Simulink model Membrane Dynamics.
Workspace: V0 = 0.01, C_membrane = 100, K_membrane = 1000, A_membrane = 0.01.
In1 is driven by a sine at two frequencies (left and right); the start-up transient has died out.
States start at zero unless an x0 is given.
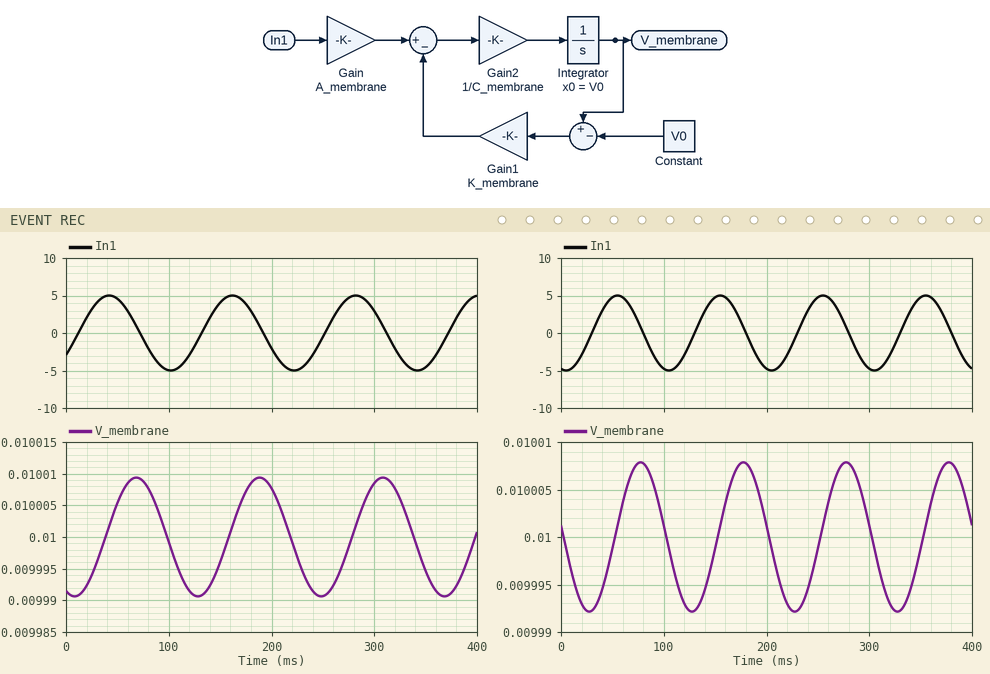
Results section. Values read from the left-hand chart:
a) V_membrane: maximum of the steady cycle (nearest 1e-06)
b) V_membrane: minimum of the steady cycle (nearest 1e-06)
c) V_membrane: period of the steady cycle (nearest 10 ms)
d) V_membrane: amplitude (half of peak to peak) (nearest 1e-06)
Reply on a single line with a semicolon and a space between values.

0.010009; 0.009991; 120 ms; 0.000009
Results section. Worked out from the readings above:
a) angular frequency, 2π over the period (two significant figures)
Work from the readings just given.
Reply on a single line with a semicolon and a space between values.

0.052 rad/ms
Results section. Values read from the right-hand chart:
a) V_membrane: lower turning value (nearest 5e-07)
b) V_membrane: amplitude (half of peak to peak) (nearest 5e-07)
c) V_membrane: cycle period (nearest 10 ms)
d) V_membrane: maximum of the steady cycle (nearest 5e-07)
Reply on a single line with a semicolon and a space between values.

0.0099920; 0.0000080; 100 ms; 0.0100080
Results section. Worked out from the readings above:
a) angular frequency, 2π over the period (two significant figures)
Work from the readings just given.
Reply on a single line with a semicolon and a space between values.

0.063 rad/ms
